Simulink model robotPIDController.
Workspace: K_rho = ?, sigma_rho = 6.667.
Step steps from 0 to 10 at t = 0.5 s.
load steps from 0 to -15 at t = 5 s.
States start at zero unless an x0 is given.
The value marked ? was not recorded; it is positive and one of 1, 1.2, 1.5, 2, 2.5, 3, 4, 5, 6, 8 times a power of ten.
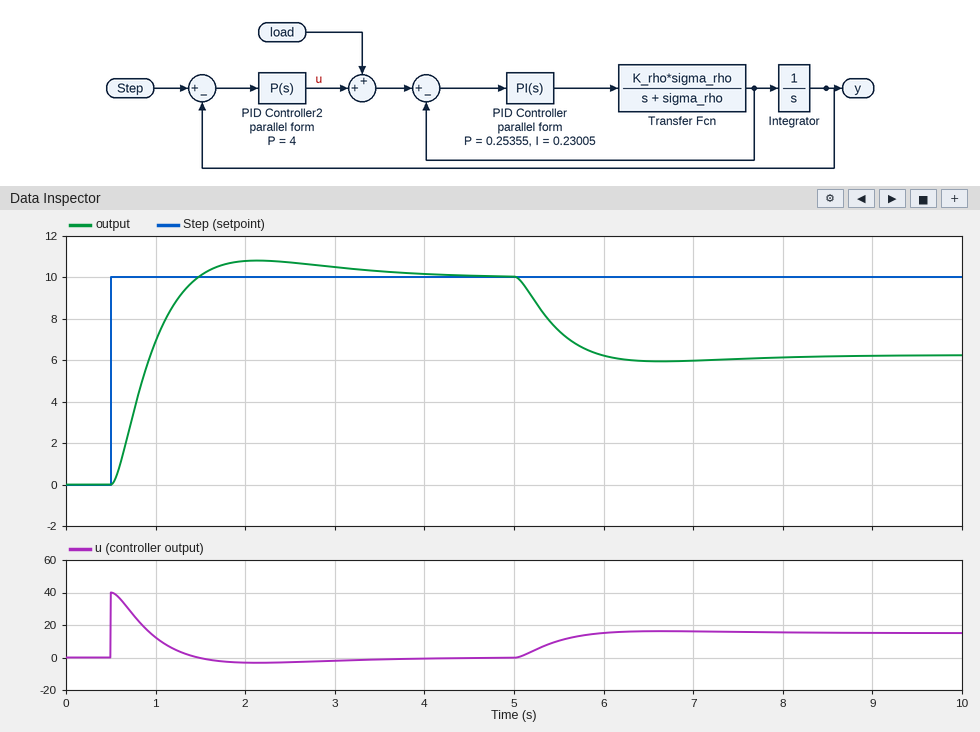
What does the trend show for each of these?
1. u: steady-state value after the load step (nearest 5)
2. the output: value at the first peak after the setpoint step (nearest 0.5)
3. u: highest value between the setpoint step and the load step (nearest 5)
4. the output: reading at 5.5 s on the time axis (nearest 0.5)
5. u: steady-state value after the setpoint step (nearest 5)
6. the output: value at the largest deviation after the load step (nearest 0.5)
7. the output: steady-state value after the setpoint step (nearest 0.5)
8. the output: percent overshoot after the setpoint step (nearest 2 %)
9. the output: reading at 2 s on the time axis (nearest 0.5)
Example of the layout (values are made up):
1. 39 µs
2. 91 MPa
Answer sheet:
1. 15
2. 11.0
3. 40
4. 7.5
5. 0
6. 6.0
7. 10.0
8. 8 %
9. 11.0
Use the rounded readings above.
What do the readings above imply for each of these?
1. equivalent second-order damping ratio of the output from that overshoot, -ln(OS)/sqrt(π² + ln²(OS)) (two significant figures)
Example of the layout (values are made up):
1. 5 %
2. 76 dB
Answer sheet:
1. 0.63
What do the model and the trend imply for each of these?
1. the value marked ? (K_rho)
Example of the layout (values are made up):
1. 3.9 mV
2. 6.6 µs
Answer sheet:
1. 4
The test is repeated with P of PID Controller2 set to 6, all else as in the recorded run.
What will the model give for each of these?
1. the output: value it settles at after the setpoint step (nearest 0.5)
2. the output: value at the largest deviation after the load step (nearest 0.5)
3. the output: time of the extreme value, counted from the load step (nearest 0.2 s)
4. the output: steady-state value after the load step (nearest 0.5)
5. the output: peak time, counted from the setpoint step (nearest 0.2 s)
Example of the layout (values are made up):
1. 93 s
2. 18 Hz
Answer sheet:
1. 10.0
2. 7.5
3. 1.2 s
4. 7.5
5. 1.2 s
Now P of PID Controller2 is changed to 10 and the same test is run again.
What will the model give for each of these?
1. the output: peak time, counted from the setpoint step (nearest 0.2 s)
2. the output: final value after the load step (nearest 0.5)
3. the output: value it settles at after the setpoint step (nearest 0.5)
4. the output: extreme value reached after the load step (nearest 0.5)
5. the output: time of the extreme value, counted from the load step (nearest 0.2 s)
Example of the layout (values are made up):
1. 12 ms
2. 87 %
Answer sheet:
1. 0.6 s
2. 8.5
3. 10.0
4. 8.5
5. 0.6 s
